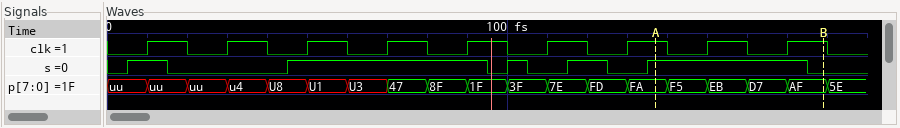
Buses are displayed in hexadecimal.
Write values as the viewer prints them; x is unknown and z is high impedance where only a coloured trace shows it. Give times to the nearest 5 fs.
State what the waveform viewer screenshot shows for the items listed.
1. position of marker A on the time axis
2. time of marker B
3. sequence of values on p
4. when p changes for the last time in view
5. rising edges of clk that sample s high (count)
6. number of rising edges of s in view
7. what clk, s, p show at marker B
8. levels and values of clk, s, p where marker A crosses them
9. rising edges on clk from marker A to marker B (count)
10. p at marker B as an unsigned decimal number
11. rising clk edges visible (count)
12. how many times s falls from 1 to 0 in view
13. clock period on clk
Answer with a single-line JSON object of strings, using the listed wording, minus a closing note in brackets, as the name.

{"position of marker A on the time axis": "135 fs", "time of marker B": "180 fs", "sequence of values on p": "uu, uu, uu, u4, U8, U1, U3, 47, 8F, 1F, 3F, 7E, FD, FA, F5, EB, D7, AF, 5E", "when p changes for the last time in view": "180 fs", "rising edges of clk that sample s high": "6", "number of rising edges of s in view": "5", "what clk, s, p show at marker B": "clk=1, s=0, p=AF", "levels and values of clk, s, p where marker A crosses them": "clk=1, s=1, p=FA", "rising edges on clk from marker A to marker B": "2", "p at marker B as an unsigned decimal number": "175", "rising clk edges visible": "9", "how many times s falls from 1 to 0 in view": "5", "clock period on clk": "20 fs"}
